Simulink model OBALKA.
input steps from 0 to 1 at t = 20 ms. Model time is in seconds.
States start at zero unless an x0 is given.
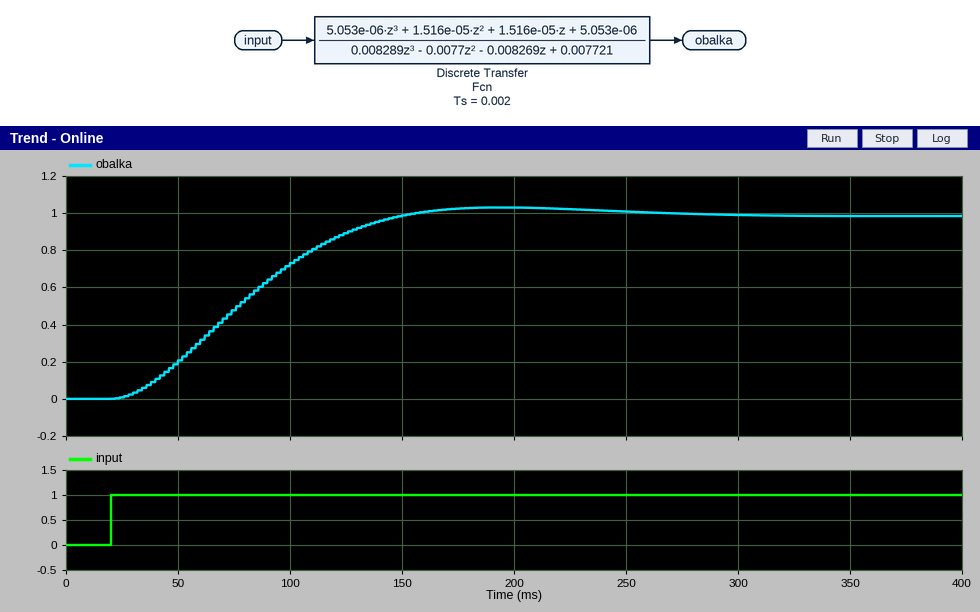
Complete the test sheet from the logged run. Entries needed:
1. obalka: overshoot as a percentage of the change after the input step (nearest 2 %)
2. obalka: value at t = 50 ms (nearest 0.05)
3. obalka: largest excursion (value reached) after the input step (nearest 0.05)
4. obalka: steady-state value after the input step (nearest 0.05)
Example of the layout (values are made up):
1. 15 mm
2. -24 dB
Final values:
1. 4 %
2. 0.20
3. 1.05
4. 1.00
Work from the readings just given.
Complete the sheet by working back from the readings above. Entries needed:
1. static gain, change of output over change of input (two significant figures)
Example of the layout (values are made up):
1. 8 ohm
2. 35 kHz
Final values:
1. 1.0
